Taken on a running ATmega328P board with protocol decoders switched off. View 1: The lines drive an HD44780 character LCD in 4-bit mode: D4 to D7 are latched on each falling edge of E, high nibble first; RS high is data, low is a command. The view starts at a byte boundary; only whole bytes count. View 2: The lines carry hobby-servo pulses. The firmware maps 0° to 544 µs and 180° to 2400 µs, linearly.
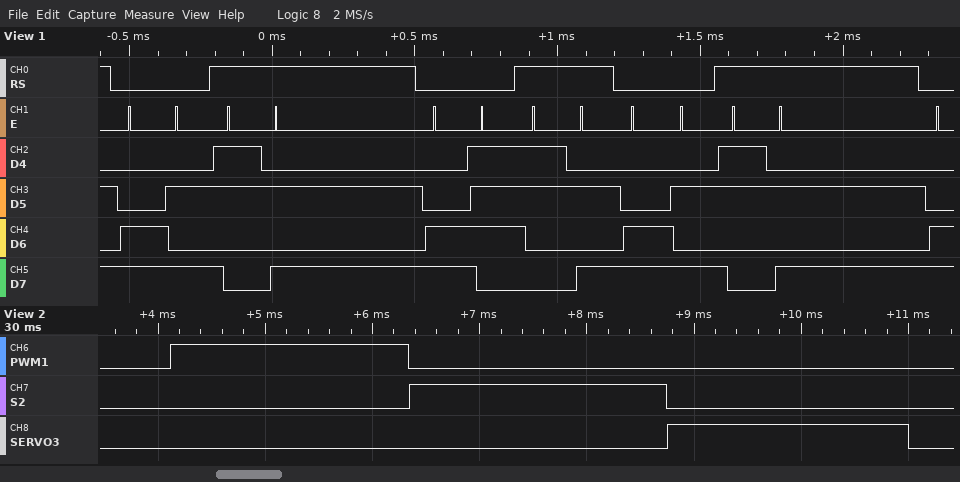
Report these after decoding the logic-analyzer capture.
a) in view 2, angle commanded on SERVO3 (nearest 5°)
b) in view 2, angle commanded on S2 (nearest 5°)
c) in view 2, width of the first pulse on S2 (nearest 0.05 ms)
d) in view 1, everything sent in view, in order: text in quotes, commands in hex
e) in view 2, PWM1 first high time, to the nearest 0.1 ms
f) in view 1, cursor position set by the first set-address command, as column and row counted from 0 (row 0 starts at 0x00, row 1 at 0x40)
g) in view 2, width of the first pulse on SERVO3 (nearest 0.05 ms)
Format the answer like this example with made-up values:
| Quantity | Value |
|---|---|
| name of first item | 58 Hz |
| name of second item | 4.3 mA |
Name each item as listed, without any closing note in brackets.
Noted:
| Quantity | Value |
|---|---|
| in view 2, angle commanded on SERVO3 | 165° |
| in view 2, angle commanded on S2 | 180° |
| in view 2, width of the first pulse on S2 | 2.40 ms |
| in view 1, everything sent in view, in order: text in quotes, commands in hex | 0xCA ":" 0xC7 ":" 0xCA ":" |
| in view 2, PWM1 first high time, to the nearest 0.1 ms | 2.2 ms |
| in view 1, cursor position set by the first set-address command, as column and row counted from 0 | column 10, row 1 |
| in view 2, width of the first pulse on SERVO3 | 2.25 ms |
